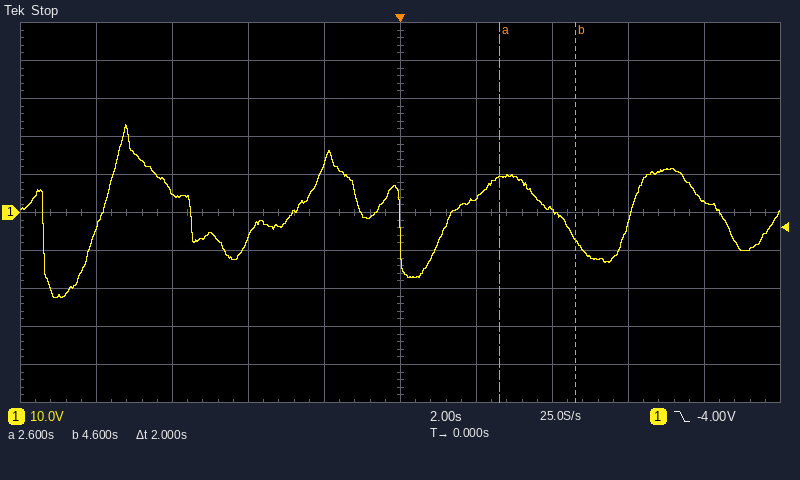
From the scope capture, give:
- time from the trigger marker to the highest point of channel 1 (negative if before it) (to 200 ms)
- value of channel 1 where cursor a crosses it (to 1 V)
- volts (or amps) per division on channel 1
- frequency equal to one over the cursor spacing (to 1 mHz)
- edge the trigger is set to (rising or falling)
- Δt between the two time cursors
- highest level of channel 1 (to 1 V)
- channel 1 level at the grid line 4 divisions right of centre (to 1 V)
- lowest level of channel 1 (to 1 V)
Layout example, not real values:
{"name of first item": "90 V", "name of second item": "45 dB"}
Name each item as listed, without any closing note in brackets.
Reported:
{"time from the trigger marker to the highest point of channel 1 (negative if before it)": "-7.2 s", "value of channel 1 where cursor a crosses it": "9 V", "volts (or amps) per division on channel 1": "10 V", "frequency equal to one over the cursor spacing": "500 mHz", "edge the trigger is set to": "falling", "Δt between the two time cursors": "2 s", "highest level of channel 1": "23 V", "channel 1 level at the grid line 4 divisions right of centre": "3 V", "lowest level of channel 1": "-22 V"}
